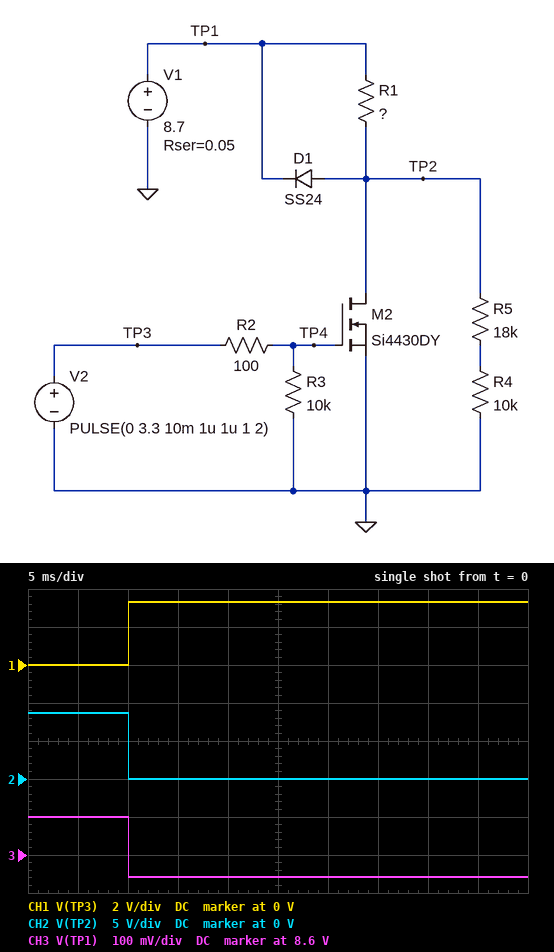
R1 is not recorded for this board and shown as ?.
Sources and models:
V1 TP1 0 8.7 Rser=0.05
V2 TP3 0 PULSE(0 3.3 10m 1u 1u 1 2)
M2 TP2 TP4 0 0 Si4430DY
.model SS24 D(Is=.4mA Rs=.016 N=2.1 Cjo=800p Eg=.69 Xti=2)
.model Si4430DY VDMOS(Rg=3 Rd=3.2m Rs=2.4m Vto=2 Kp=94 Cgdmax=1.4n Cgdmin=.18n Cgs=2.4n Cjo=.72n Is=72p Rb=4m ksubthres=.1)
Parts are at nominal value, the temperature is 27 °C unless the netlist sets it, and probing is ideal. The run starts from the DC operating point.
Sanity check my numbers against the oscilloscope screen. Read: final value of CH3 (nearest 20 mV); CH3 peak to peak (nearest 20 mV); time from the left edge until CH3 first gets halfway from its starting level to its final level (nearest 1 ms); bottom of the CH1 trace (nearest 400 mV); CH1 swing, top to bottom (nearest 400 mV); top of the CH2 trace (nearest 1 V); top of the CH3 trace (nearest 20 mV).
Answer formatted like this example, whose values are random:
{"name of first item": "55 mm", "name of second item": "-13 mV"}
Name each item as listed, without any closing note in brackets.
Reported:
{"final value of CH3": "8.54 V", "CH3 peak to peak": "160 mV", "time from the left edge until CH3 first gets halfway from its starting level to its final level": "10 ms", "bottom of the CH1 trace": "0 V", "CH1 swing, top to bottom": "3.2 V", "top of the CH2 trace": "9 V", "top of the CH3 trace": "8.70 V"}
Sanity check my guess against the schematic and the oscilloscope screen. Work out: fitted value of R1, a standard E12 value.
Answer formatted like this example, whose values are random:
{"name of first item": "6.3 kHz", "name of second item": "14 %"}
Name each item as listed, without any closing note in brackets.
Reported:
{"fitted value of R1, a standard E12 value": "2.7 Ω"}
